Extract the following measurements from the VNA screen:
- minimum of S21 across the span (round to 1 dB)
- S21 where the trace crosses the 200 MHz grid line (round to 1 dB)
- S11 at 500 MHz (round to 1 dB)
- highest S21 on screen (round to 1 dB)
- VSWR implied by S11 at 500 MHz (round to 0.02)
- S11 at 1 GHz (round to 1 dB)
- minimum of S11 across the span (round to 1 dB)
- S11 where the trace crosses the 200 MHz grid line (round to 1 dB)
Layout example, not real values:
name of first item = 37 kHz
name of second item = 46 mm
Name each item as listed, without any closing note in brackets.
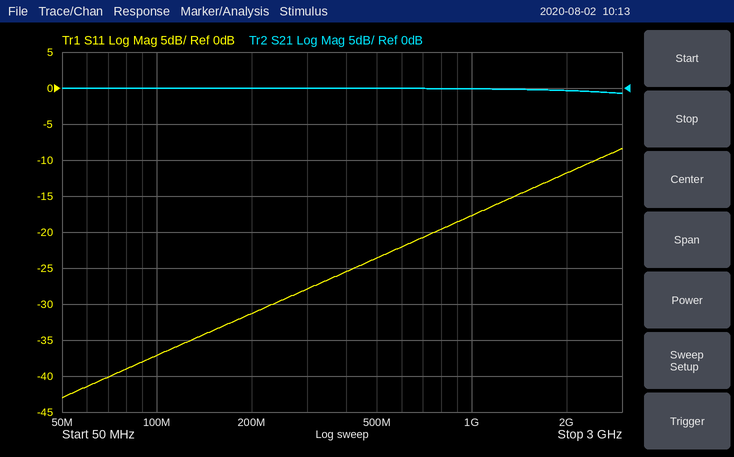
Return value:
minimum of S21 across the span = -1 dB
S21 where the trace crosses the 200 MHz grid line = 0 dB
S11 at 500 MHz = -24 dB
highest S21 on screen = 0 dB
VSWR implied by S11 at 500 MHz = 1.14
S11 at 1 GHz = -18 dB
minimum of S11 across the span = -43 dB
S11 where the trace crosses the 200 MHz grid line = -31 dB
